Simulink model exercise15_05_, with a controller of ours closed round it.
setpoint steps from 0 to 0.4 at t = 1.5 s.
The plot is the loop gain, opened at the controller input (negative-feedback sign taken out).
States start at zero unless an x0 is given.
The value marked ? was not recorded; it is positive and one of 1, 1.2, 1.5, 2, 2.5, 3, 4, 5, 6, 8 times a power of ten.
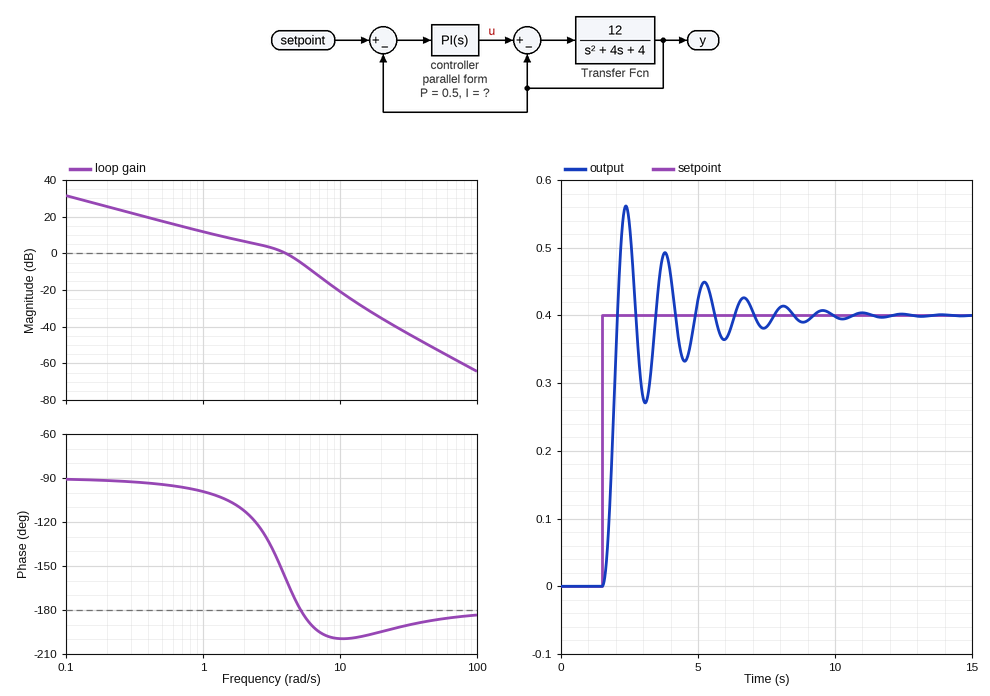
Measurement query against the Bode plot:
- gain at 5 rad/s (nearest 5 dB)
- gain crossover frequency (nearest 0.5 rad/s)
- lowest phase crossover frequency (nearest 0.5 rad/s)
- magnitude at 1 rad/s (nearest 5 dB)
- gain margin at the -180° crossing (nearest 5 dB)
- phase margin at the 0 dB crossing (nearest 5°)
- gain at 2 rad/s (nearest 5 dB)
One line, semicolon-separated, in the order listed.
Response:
-5 dB; 4.0 rad/s; 5.0 rad/s; 10 dB; 5 dB; 20°; 5 dB
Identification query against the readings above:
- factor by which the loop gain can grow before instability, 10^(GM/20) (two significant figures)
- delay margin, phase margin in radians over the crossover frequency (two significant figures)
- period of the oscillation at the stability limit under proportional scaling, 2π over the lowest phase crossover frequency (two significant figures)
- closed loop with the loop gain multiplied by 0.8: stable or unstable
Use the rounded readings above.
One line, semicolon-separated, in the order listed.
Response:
1.8; 0.087 s; 1.3 s; stable
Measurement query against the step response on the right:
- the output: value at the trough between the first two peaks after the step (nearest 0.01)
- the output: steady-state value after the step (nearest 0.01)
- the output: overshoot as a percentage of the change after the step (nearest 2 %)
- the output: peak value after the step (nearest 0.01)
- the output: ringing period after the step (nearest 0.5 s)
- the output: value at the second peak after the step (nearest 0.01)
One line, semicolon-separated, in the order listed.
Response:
0.27; 0.40; 40 %; 0.56; 1.5 s; 0.49
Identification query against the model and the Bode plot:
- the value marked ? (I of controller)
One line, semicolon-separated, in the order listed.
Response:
5
